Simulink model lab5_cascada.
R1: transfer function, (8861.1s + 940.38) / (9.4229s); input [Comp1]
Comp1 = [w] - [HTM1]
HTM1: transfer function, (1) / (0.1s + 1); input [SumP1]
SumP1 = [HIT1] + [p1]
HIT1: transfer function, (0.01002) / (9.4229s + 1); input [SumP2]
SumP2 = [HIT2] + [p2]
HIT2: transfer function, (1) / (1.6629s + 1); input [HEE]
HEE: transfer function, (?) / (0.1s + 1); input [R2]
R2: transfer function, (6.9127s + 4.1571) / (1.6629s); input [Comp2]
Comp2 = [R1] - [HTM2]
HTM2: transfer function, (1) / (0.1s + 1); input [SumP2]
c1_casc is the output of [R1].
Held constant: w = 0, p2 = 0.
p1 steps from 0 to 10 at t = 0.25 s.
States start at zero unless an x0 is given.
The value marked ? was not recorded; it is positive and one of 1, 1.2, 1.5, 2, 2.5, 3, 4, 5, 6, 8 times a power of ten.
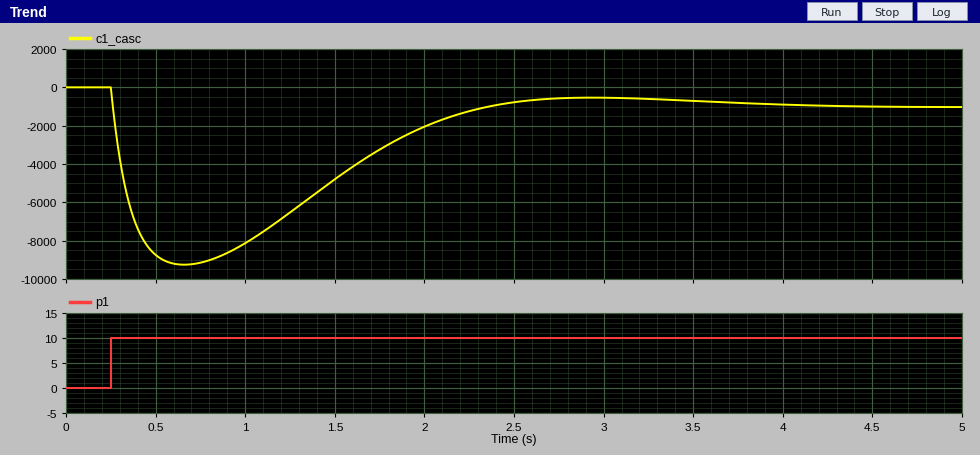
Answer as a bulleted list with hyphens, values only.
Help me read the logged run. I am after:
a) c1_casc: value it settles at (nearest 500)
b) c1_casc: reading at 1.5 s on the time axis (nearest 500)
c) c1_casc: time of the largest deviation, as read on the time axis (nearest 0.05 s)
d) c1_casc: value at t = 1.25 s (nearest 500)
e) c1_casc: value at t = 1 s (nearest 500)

- -1000
- -5000
- 0.65 s
- -6500
- -8000
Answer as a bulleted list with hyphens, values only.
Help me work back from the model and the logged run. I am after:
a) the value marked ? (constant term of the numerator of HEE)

- 0.8
